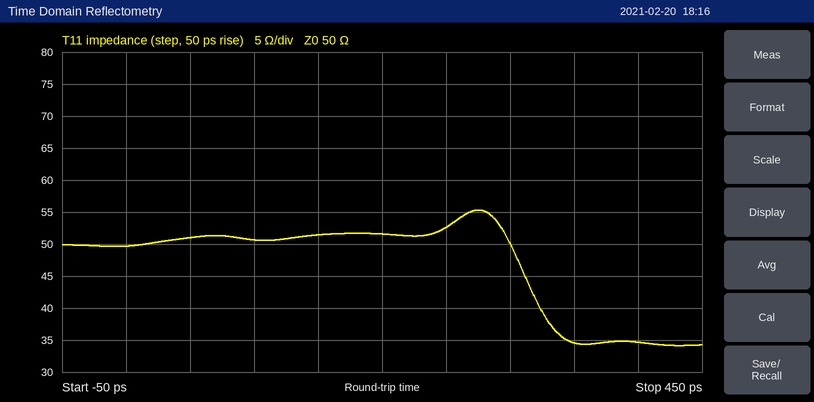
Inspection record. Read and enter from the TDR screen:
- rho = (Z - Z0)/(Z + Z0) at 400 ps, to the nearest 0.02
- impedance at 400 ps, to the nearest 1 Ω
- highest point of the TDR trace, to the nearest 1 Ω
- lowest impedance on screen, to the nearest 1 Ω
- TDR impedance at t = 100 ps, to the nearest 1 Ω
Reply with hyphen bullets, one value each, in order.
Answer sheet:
- -0.18
- 35 Ω
- 55 Ω
- 34 Ω
- 51 Ω
